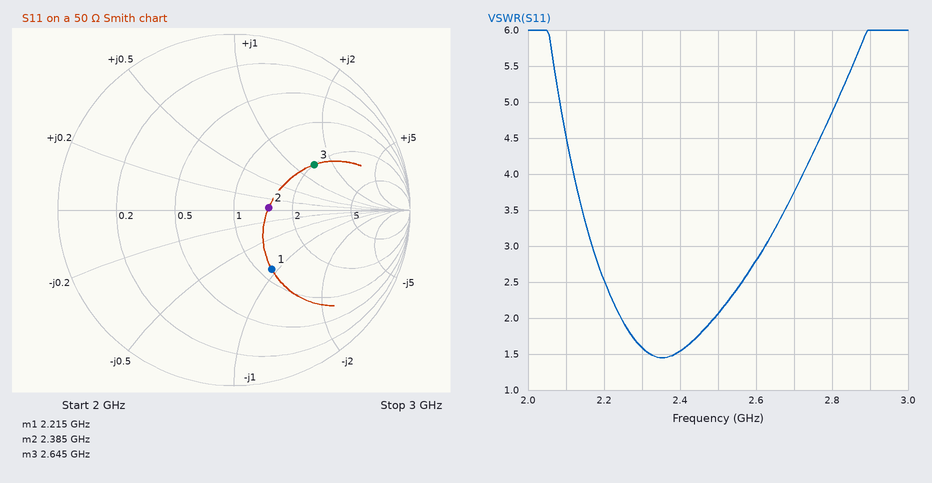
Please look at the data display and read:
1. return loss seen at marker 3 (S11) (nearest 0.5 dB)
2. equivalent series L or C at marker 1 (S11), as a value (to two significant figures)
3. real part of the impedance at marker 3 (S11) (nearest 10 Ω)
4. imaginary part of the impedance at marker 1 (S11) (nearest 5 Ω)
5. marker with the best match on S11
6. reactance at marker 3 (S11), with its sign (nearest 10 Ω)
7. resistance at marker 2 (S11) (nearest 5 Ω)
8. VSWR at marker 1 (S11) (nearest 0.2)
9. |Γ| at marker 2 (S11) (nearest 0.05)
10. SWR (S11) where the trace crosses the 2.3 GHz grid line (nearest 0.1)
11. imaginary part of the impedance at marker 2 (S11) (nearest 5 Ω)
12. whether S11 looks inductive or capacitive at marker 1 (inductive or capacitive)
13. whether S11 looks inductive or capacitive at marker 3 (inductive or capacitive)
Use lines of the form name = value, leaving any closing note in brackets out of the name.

return loss seen at marker 3 (S11) = 5.5 dB
equivalent series L or C at marker 1 (S11), as a value = 1.6 pF
real part of the impedance at marker 3 (S11) = 100 Ω
imaginary part of the impedance at marker 1 (S11) = -45 Ω
marker with the best match on S11 = marker 2
reactance at marker 3 (S11), with its sign = +70 Ω
resistance at marker 2 (S11) = 75 Ω
VSWR at marker 1 (S11) = 2.4
|Γ| at marker 2 (S11) = 0.20
SWR (S11) where the trace crosses the 2.3 GHz grid line = 1.6
imaginary part of the impedance at marker 2 (S11) = 0 Ω
whether S11 looks inductive or capacitive at marker 1 = capacitive
whether S11 looks inductive or capacitive at marker 3 = inductive
